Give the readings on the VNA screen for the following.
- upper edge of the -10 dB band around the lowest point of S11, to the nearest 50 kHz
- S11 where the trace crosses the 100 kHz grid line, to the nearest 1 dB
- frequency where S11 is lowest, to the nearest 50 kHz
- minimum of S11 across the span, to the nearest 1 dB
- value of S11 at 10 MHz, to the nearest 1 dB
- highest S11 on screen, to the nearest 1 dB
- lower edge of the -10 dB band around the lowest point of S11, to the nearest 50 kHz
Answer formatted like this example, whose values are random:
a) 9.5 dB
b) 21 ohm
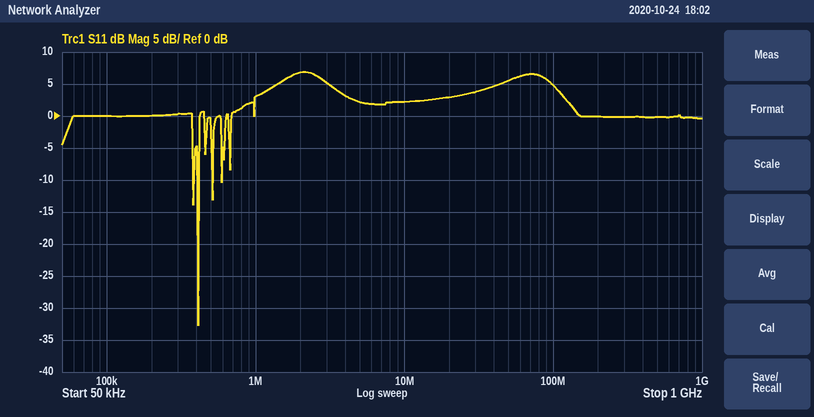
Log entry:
a) 400 kHz
b) 0 dB
c) 400 kHz
d) -33 dB
e) 2 dB
f) 7 dB
g) 400 kHz
